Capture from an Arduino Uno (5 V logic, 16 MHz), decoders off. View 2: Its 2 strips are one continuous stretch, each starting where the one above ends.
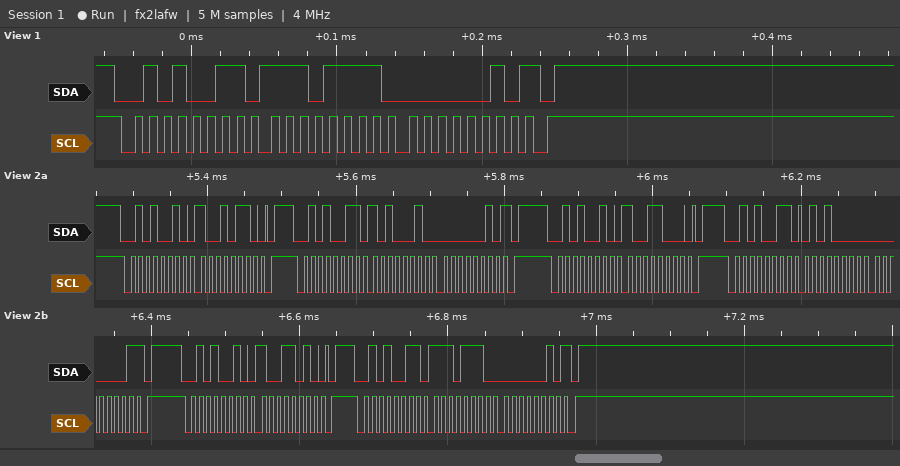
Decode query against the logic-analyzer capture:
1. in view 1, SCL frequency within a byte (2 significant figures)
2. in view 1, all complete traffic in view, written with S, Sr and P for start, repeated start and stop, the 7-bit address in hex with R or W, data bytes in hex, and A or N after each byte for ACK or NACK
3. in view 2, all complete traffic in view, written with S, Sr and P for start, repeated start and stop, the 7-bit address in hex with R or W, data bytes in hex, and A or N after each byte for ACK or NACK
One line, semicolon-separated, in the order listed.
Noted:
100 kHz; S 29R A EF A 02 N P; S 29W A 96 A P S 29R A A2 A 02 N P S 29W A 98 A P S 29R A 50 A 01 N P S 29W A 9A A P S 29R A EE A 02 N P
